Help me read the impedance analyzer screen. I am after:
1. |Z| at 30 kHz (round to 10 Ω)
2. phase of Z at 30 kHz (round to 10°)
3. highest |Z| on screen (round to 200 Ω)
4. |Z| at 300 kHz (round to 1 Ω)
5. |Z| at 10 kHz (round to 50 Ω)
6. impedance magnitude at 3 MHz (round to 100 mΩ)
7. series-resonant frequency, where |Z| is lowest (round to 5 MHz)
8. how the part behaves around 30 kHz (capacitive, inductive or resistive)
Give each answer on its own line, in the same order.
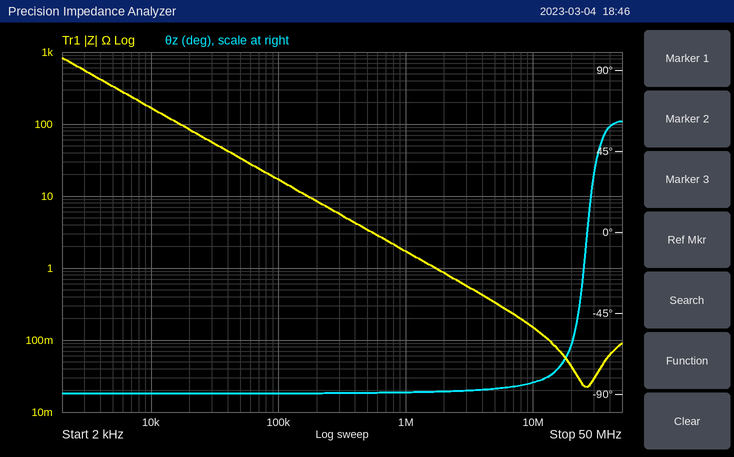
60 Ω
-90°
800 Ω
6 Ω
150 Ω
600 mΩ
25 MHz
capacitive
